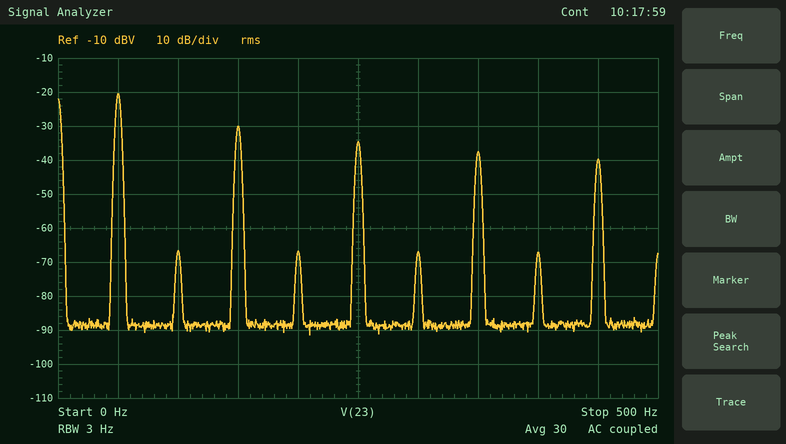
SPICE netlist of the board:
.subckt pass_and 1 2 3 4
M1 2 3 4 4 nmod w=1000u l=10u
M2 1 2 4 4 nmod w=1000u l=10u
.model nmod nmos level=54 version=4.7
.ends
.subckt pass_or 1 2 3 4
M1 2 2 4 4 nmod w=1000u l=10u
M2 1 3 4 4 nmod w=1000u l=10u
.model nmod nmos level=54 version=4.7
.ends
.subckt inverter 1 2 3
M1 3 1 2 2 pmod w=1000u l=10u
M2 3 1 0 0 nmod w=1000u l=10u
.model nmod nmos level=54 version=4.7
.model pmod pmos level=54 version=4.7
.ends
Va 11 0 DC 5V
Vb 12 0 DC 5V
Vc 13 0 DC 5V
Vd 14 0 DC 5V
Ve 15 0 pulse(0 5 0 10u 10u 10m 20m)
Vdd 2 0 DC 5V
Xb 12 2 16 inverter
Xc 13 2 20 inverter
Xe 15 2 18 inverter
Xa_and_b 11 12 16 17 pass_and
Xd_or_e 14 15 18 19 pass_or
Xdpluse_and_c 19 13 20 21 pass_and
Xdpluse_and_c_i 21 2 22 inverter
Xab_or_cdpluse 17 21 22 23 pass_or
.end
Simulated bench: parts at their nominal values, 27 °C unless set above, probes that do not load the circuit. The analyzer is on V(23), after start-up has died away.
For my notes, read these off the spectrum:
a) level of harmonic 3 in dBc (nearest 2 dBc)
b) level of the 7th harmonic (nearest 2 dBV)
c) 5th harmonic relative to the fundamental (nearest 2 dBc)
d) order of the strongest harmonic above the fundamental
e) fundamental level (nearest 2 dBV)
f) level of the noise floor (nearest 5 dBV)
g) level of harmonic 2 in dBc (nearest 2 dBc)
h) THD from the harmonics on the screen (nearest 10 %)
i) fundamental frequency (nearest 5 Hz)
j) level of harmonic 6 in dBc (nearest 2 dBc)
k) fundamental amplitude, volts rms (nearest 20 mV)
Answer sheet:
-10 dBc
-38 dBV
-14 dBc
3
-20 dBV
-90 dBV
-46 dBc
40 %
50 Hz
-46 dBc
100 mV
